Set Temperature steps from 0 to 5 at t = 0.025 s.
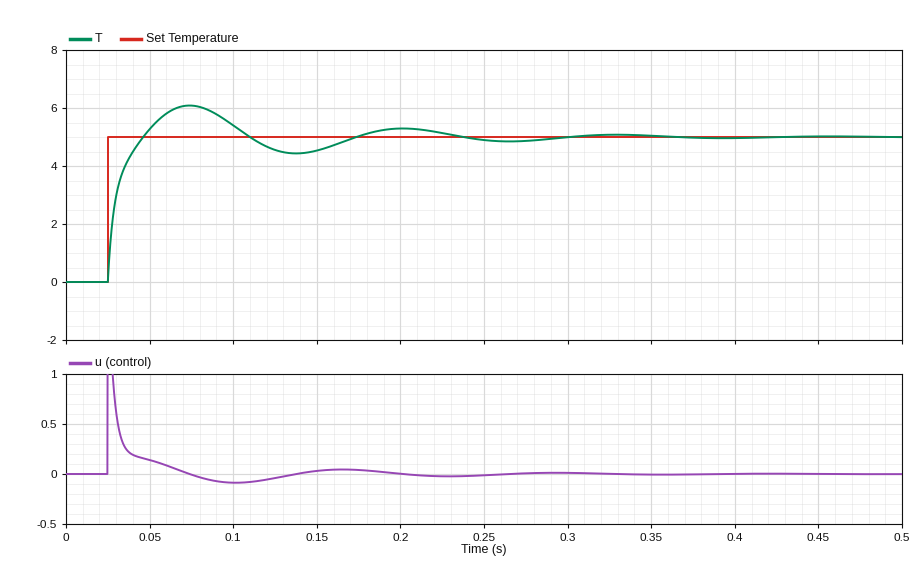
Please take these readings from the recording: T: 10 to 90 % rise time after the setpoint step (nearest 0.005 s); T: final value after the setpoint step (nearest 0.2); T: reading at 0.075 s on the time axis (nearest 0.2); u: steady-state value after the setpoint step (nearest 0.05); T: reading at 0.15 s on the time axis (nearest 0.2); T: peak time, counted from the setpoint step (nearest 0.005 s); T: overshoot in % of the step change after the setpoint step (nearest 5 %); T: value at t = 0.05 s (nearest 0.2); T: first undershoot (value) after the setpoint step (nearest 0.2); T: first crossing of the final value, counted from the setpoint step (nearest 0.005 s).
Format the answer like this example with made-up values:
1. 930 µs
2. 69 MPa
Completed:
1. 0.015 s
2. 5.0
3. 6.0
4. 0.00
5. 4.6
6. 0.050 s
7. 20 %
8. 5.2
9. 4.4
10. 0.020 s
